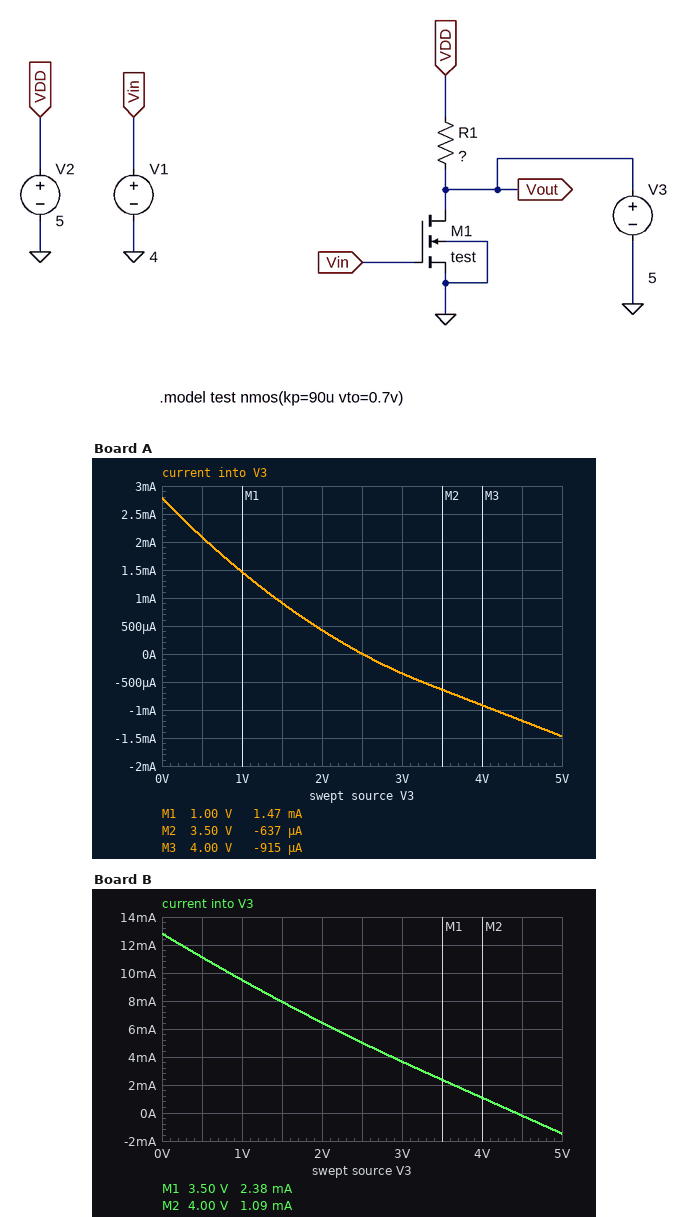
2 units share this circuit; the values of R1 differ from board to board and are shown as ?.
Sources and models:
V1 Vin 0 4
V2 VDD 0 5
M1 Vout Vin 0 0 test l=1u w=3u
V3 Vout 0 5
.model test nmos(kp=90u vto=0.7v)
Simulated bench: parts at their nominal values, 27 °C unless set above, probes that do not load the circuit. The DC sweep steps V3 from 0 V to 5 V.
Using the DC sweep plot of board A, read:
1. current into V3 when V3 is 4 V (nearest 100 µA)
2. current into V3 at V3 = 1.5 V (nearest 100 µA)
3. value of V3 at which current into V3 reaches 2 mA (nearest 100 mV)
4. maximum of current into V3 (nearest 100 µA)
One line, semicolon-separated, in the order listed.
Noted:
-900 µA; 900 µA; 600 mV; 2.8 mA
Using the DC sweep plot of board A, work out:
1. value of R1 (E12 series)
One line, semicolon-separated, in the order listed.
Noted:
1.8 kΩ
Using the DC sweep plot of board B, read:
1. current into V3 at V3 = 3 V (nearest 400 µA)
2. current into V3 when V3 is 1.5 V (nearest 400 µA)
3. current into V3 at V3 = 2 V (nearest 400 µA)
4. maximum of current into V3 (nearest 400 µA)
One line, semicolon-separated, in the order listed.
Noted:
3.6 mA; 8.0 mA; 6.4 mA; 12.8 mA
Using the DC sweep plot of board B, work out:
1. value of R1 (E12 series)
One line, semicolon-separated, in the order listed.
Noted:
390 Ω
